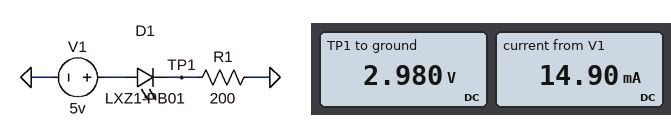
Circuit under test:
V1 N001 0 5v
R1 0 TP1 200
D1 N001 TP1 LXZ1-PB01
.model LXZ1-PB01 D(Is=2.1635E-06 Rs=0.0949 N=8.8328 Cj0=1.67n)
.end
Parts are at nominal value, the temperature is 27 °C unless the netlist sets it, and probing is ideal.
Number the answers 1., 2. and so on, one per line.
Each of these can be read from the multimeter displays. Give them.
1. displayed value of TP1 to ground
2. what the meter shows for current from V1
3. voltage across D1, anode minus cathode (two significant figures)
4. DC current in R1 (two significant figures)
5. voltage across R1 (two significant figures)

1. 2.980 V
2. 14.90 mA
3. 2.0 V
4. 15 mA
5. 3.0 V
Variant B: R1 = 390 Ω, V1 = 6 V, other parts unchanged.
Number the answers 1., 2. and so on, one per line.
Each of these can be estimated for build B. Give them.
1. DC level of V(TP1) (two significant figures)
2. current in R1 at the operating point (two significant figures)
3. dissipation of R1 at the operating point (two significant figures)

1. 4.1 V
2. 10 mA
3. 42 mW
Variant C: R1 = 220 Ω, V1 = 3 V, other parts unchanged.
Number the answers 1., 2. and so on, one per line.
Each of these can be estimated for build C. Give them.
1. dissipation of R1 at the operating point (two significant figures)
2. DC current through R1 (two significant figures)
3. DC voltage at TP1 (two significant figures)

1. 6.6 mW
2. 5.5 mA
3. 1.2 V
